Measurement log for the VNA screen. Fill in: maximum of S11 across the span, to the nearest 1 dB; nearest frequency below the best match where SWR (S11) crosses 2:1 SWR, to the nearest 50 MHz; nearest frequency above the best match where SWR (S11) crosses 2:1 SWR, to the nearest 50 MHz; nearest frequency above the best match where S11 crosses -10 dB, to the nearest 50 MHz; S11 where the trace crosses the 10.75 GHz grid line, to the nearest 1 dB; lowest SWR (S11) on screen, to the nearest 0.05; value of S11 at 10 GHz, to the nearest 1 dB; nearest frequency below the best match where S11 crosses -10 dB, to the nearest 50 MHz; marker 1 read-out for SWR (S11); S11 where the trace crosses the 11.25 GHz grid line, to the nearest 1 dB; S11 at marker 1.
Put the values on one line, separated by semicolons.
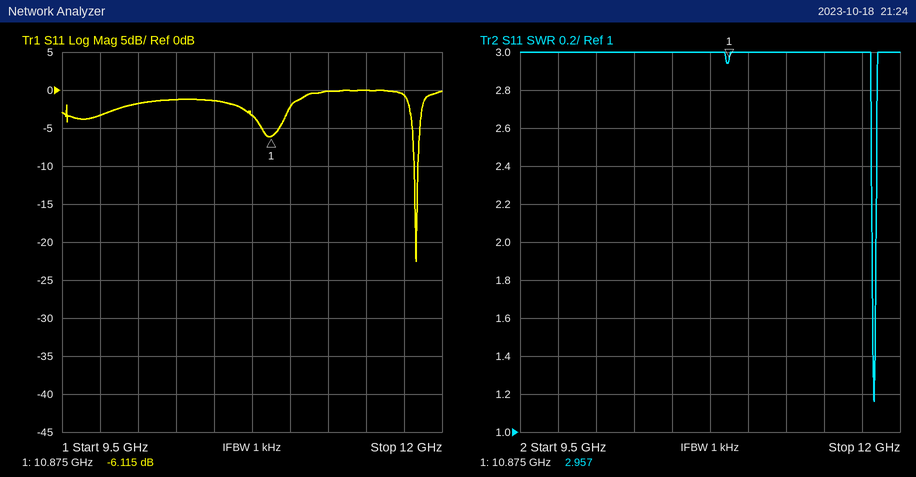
0 dB; 11.80 GHz; 11.85 GHz; 11.85 GHz; -3 dB; 1.15; -2 dB; 11.80 GHz; 2.957; 0 dB; -6.115 dB
